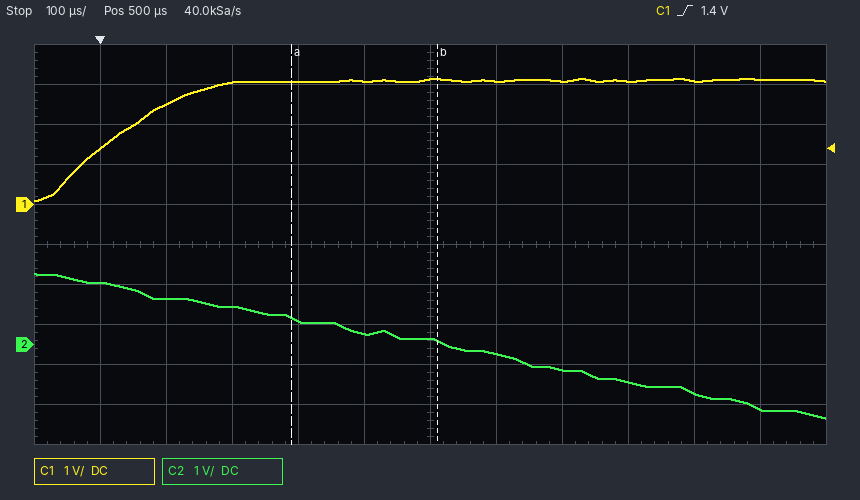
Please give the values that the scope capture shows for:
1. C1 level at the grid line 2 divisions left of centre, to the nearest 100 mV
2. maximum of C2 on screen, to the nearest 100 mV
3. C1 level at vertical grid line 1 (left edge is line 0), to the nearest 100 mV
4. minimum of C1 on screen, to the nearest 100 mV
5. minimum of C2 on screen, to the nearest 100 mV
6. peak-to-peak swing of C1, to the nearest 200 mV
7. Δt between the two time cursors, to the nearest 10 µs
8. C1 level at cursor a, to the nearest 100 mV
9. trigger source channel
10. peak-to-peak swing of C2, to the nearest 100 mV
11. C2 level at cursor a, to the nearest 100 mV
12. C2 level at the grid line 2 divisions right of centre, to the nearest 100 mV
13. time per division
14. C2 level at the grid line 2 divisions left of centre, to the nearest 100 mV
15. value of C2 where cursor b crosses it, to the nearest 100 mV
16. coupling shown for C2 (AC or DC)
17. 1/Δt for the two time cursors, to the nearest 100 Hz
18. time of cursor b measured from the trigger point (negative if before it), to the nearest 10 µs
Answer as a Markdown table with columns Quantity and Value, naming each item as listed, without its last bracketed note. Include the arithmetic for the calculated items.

| Quantity | Value |
|---|---|
| C1 level at the grid line 2 divisions left of centre, to the nearest 100 mV | 3.1 V |
| maximum of C2 on screen, to the nearest 100 mV | 1.8 V |
| C1 level at vertical grid line 1 (left edge is line 0), to the nearest 100 mV | 1.4 V |
| minimum of C1 on screen, to the nearest 100 mV | 100 mV |
| minimum of C2 on screen, to the nearest 100 mV | -1.8 V |
| peak-to-peak swing of C1, to the nearest 200 mV | 3.0 V |
| Δt between the two time cursors, to the nearest 10 µs | 220 µs |
| C1 level at cursor a, to the nearest 100 mV | 3.1 V |
| trigger source channel | C1 |
| peak-to-peak swing of C2, to the nearest 100 mV | 1.8 V − (-1.8 V) = 3.6 V |
| C2 level at cursor a, to the nearest 100 mV | 700 mV |
| C2 level at the grid line 2 divisions right of centre, to the nearest 100 mV | -600 mV |
| time per division | 100 µs |
| C2 level at the grid line 2 divisions left of centre, to the nearest 100 mV | 600 mV |
| value of C2 where cursor b crosses it, to the nearest 100 mV | 100 mV |
| coupling shown for C2 | DC |
| 1/Δt for the two time cursors, to the nearest 100 Hz | 1 / 220 µs ≈ 4.5 kHz |
| time of cursor b measured from the trigger point (negative if before it), to the nearest 10 µs | +510 µs |
